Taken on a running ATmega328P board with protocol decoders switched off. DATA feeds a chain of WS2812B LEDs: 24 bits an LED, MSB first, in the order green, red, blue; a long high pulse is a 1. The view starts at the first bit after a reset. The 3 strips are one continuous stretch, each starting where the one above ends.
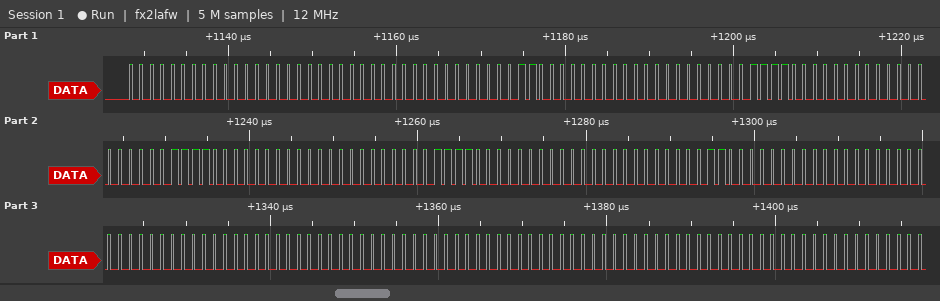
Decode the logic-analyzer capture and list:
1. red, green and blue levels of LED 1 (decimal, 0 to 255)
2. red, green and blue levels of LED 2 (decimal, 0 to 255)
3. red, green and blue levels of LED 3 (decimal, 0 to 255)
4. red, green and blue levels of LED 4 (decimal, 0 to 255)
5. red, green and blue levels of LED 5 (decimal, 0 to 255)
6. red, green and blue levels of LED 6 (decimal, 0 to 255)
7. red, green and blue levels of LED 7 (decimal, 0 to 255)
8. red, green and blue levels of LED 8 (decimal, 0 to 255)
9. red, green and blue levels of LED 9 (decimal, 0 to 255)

0, 0, 0
6, 0, 0
30, 0, 0
60, 0, 0
30, 0, 0
6, 0, 0
0, 0, 0
0, 0, 0
0, 0, 0
